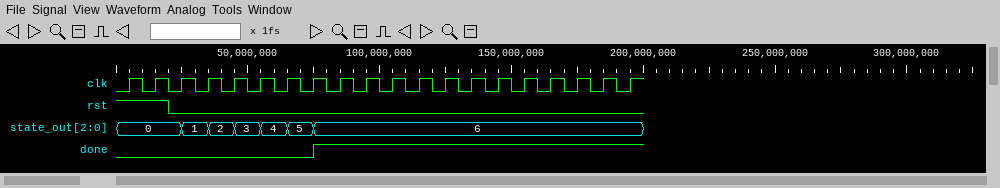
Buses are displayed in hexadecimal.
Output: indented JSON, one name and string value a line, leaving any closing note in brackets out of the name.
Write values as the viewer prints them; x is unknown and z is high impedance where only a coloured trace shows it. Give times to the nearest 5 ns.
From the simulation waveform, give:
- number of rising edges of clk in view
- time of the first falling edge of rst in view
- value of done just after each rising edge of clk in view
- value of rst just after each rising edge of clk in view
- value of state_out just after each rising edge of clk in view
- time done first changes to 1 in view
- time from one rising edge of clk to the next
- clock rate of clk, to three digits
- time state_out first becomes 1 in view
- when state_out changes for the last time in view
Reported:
{
  "number of rising edges of clk in view": "20",
  "time of the first falling edge of rst in view": "20 ns",
  "value of done just after each rising edge of clk in view": "0 0 0 0 0 0 0 1 1 1 1 1 1 1 1 1 1 1 1 1",
  "value of rst just after each rising edge of clk in view": "1 1 0 0 0 0 0 0 0 0 0 0 0 0 0 0 0 0 0 0",
  "value of state_out just after each rising edge of clk in view": "0, 0, 1, 2, 3, 4, 5, 6, 6, 6, 6, 6, 6, 6, 6, 6, 6, 6, 6, 6",
  "time done first changes to 1 in view": "75 ns",
  "time from one rising edge of clk to the next": "10 ns",
  "clock rate of clk, to three digits": "100 MHz",
  "time state_out first becomes 1 in view": "25 ns",
  "when state_out changes for the last time in view": "75 ns"
}
